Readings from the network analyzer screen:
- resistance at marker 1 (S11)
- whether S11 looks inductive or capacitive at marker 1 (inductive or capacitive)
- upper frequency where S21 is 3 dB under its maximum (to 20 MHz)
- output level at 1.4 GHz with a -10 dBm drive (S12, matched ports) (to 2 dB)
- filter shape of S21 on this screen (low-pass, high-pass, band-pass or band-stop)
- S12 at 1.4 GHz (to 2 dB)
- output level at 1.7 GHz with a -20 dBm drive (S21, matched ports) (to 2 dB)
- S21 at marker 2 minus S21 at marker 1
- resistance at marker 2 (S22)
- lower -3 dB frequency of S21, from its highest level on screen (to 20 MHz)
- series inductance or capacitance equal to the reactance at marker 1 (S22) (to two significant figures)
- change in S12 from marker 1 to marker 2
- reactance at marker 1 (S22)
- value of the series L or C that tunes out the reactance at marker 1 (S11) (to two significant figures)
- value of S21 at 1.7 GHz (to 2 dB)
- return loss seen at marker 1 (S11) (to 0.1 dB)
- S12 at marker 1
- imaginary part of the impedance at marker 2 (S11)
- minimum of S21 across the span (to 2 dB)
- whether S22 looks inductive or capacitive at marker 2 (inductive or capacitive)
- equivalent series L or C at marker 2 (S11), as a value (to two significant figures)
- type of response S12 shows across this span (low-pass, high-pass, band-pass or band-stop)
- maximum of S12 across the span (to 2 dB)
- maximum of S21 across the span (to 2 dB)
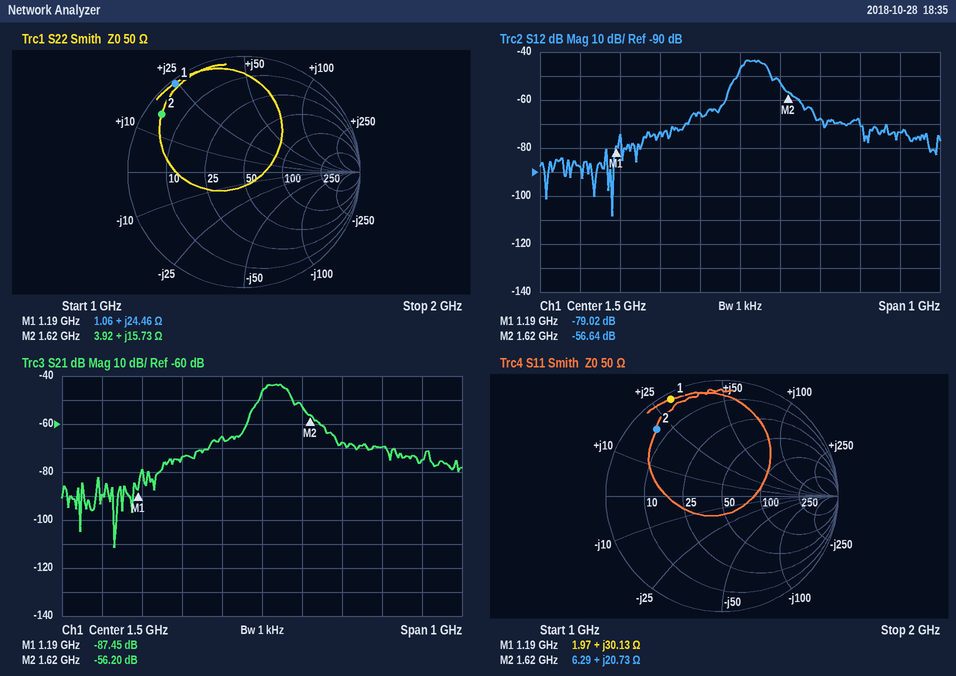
1.97 Ω
inductive
1.56 GHz
-76 dBm
band-pass
-66 dB
-88 dBm
31.25 dB
3.92 Ω
1.50 GHz
3.3 nH
22.38 dB
+24.46 Ω
4.4 pF
-68 dB
0.5 dB
-79.02 dB
+20.73 Ω
-112 dB
inductive
2.0 nH
band-pass
-44 dB
-44 dB
